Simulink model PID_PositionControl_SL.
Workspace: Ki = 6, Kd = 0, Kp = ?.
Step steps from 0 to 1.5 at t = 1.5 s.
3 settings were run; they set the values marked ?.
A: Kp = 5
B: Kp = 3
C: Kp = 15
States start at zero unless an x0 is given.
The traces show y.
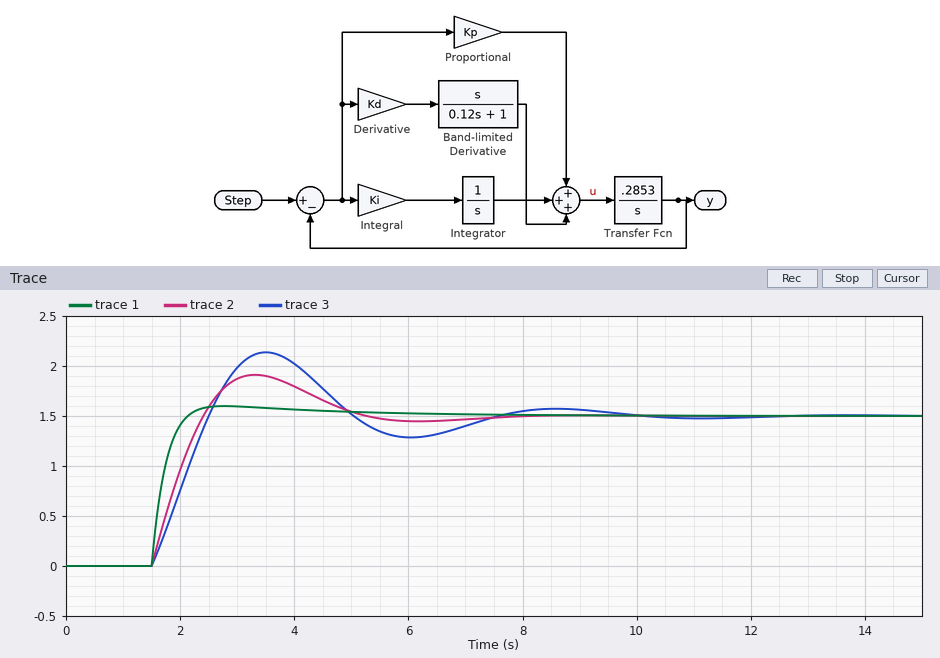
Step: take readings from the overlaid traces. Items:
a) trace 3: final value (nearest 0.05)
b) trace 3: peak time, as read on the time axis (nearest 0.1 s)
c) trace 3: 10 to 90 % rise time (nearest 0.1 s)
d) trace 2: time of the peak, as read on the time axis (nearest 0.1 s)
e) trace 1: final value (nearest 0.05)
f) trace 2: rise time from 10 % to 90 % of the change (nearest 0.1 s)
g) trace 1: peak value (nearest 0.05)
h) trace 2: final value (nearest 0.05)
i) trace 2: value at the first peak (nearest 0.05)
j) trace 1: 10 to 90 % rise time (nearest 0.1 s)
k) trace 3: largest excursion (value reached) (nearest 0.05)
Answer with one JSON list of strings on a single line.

["1.50", "3.5 s", "0.8 s", "3.3 s", "1.50", "0.7 s", "1.60", "1.50", "1.90", "0.4 s", "2.15"]
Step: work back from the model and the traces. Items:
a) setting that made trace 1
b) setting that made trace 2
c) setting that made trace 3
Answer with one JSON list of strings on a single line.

["C", "A", "B"]
